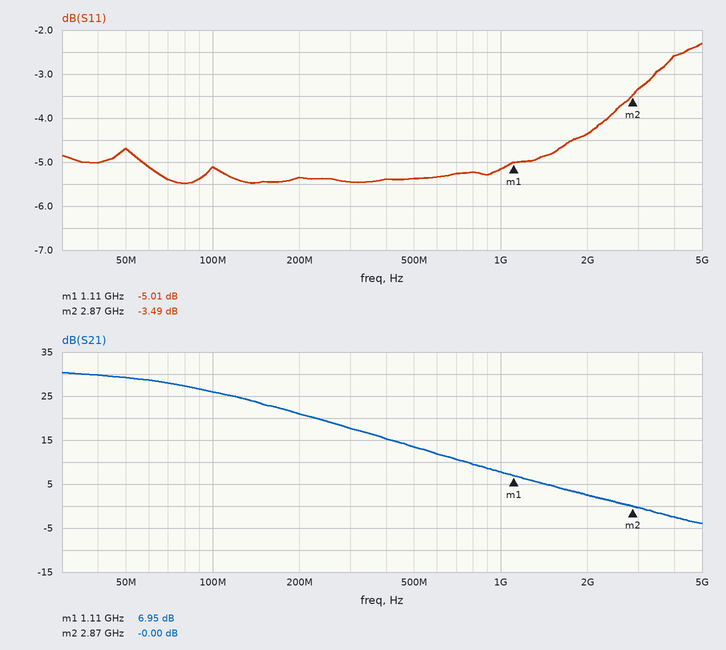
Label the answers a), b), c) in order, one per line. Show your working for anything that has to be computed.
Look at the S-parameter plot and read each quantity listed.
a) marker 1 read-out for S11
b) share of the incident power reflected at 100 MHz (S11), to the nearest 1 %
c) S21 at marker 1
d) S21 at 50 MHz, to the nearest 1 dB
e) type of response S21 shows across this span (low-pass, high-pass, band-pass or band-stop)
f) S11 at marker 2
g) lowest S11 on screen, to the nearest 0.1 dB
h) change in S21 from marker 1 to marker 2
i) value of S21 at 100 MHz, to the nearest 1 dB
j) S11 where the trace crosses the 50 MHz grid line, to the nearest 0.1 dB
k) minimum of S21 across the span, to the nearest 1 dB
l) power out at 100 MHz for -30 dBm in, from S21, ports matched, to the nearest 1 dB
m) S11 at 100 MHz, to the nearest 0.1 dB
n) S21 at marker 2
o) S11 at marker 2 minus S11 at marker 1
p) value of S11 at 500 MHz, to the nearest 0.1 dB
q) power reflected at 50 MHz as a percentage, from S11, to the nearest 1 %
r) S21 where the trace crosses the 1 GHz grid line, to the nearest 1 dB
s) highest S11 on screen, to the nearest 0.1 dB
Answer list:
a) -5.01 dB
b) 10^(-5.1/10) ≈ 31 %
c) 6.95 dB
d) 29 dB
e) low-pass
f) -3.49 dB
g) -5.5 dB
h) -0 − (6.95) = -6.95 dB
i) 26 dB
j) -4.7 dB
k) -4 dB
l) -30 dBm + (26 dB) = -4 dBm
m) -5.1 dB
n) -0.00 dB
o) -3.49 − (-5.01) = 1.52 dB
p) -5.4 dB
q) 10^(-4.7/10) ≈ 34 %
r) 8 dB
s) -2.3 dB
